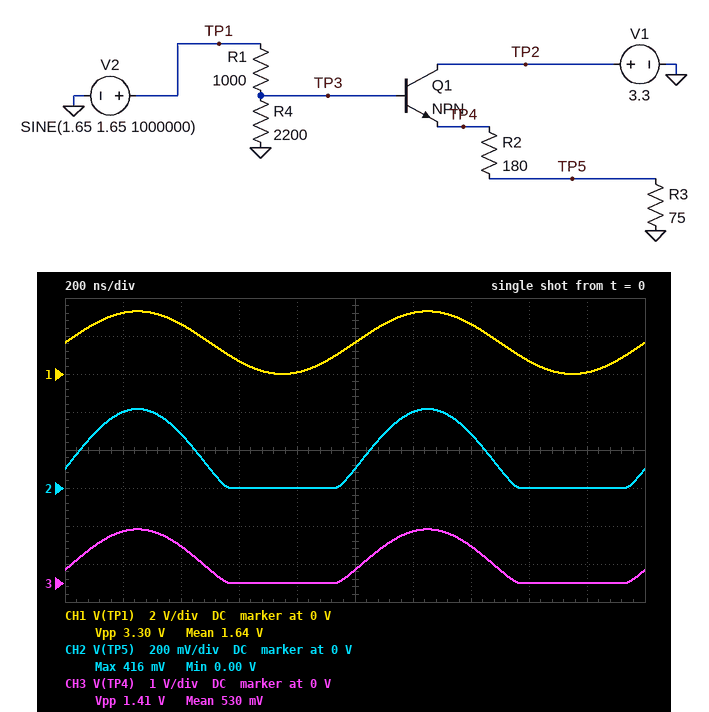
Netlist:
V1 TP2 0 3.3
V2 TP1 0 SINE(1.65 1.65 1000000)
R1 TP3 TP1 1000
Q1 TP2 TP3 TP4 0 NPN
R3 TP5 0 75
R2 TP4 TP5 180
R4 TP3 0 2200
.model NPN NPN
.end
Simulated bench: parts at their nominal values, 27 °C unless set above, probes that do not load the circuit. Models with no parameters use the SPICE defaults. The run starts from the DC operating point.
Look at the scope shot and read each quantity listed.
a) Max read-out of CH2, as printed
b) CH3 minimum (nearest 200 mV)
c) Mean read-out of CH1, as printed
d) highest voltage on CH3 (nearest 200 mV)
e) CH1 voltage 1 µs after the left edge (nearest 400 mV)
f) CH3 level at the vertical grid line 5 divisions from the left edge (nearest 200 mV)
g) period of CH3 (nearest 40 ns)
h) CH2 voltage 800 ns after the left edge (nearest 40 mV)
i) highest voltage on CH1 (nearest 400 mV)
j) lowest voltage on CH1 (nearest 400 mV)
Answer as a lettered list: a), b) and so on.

a) 416 mV
b) 0 V
c) 1.64 V
d) 1.4 V
e) 1.6 V
f) 400 mV
g) 1.00 µs
h) 0 V
i) 3.2 V
j) 0 V
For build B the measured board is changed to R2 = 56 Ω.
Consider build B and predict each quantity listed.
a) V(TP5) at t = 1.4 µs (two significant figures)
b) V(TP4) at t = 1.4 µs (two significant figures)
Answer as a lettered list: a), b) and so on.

a) 530 mV
b) 930 mV
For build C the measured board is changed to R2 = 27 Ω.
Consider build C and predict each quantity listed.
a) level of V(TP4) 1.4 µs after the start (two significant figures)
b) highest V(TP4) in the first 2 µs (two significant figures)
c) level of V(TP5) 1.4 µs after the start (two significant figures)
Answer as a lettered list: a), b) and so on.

a) 910 mV
b) 1.3 V
c) 670 mV
